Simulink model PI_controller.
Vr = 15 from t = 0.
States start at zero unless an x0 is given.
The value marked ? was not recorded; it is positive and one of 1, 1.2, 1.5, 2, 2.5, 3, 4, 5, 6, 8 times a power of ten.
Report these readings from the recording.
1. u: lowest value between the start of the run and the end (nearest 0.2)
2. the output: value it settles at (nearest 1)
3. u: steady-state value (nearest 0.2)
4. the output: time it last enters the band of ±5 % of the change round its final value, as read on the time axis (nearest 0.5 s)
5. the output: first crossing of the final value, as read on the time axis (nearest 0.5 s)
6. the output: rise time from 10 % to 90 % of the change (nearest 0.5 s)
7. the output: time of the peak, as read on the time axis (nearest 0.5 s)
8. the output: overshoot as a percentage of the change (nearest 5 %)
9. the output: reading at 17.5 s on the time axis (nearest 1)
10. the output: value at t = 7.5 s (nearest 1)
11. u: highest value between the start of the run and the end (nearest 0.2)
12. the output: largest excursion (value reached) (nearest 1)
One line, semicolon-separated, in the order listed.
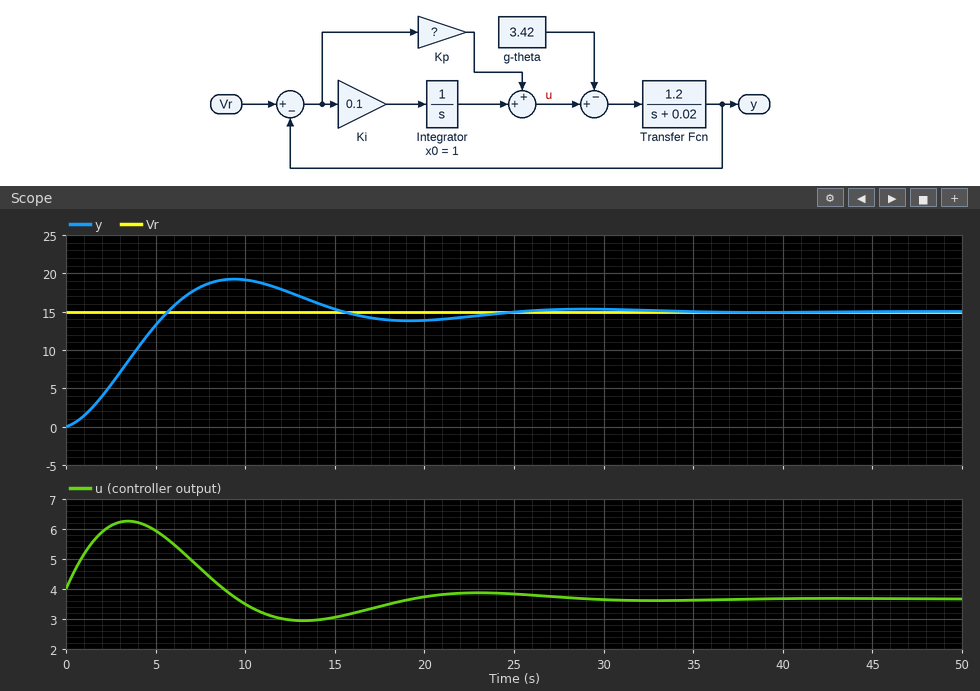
3.0; 15; 3.6; 22.0 s; 5.5 s; 4.0 s; 9.5 s; 30 %; 14; 18; 6.2; 19
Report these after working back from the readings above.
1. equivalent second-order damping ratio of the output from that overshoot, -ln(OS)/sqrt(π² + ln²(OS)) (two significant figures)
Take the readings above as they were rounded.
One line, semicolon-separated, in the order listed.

0.36
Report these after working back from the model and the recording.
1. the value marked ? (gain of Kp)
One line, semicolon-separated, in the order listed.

0.2
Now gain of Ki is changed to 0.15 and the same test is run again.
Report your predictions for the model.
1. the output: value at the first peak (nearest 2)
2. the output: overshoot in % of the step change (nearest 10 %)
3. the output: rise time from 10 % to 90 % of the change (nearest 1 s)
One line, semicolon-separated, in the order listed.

20; 40 %; 3 s
